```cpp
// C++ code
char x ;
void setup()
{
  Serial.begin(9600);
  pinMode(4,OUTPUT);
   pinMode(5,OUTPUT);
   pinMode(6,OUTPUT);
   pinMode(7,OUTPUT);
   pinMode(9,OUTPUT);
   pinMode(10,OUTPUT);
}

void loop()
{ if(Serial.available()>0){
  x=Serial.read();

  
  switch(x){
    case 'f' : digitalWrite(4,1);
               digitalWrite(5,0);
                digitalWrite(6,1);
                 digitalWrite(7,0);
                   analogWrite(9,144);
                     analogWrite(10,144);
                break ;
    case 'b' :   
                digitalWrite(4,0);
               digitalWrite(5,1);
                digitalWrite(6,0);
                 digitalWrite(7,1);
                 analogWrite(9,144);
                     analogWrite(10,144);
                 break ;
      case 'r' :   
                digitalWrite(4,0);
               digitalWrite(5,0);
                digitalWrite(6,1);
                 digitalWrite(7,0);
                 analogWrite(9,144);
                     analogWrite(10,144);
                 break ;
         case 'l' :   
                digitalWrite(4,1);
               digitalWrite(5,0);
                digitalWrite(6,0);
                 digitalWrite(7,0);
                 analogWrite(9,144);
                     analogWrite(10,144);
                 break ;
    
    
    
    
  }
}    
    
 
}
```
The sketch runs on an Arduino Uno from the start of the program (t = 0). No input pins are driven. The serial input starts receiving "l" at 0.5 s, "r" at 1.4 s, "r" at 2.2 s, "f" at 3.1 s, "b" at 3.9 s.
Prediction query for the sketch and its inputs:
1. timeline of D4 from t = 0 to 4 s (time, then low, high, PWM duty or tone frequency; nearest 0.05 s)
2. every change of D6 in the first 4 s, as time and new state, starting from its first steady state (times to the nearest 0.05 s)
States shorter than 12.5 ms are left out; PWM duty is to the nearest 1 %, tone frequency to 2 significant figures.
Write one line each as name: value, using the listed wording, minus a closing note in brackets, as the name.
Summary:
timeline of D4 from t = 0 to 4 s: 0 s low; 0.5 s high; 1.4 s low; 3.1 s high; 3.9 s low
every change of D6 in the first 4 s, as time and new state, starting from its first steady state: 0 s low; 1.4 s high; 3.9 s low
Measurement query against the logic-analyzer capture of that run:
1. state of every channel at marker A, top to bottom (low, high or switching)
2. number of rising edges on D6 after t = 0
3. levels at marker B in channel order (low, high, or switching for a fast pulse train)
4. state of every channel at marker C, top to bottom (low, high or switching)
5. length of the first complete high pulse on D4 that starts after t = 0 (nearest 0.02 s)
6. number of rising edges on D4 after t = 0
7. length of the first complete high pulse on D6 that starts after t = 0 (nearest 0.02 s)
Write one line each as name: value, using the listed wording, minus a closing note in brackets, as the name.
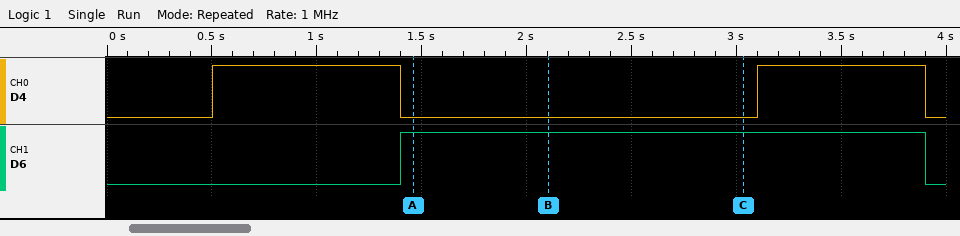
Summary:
state of every channel at marker A, top to bottom: D4 low, D6 high
number of rising edges on D6 after t = 0: 1
levels at marker B in channel order: D4 low, D6 high
state of every channel at marker C, top to bottom: D4 low, D6 high
length of the first complete high pulse on D4 that starts after t = 0: 0.90 s
number of rising edges on D4 after t = 0: 2
length of the first complete high pulse on D6 that starts after t = 0: 2.50 s
